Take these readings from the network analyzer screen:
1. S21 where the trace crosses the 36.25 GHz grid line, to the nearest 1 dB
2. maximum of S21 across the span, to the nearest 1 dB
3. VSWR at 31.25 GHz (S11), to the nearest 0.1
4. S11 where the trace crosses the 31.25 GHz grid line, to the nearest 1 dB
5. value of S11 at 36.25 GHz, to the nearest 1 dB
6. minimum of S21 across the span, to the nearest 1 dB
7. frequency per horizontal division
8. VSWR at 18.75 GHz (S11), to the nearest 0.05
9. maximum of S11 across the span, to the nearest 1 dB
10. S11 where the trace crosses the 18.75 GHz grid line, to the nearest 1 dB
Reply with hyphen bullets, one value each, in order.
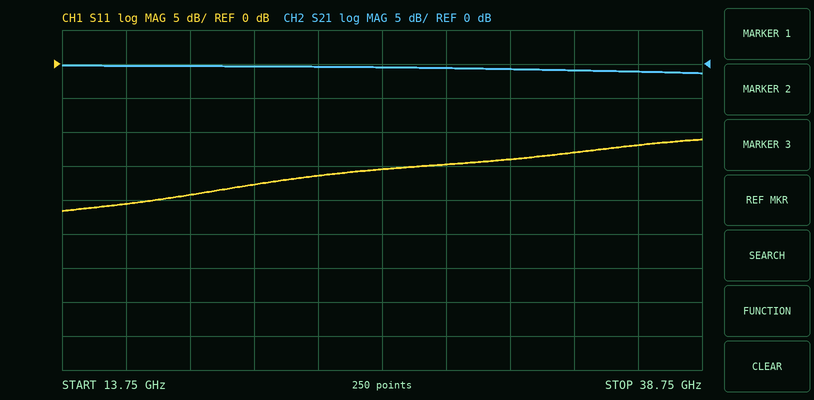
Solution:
- -1 dB
- 0 dB
- 1.5
- -14 dB
- -12 dB
- -1 dB
- 2.5 GHz
- 1.25
- -11 dB
- -19 dB
